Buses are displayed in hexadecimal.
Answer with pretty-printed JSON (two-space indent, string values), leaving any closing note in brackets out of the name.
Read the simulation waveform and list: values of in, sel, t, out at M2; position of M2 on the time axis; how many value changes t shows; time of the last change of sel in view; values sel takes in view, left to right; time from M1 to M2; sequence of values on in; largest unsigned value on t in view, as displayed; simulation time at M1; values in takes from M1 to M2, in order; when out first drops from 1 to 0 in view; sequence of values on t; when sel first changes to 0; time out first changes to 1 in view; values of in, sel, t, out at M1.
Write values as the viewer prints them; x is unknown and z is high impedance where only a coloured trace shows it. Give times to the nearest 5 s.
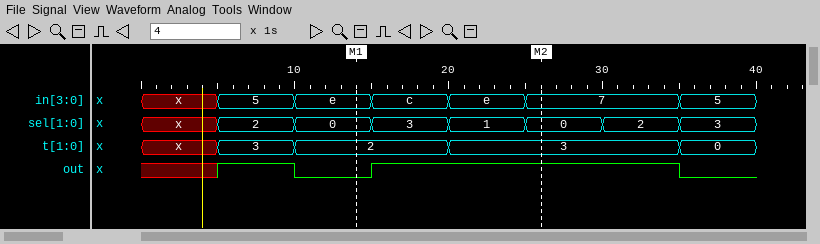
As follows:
{
  "values of in, sel, t, out at M2": "in=7, sel=0, t=3, out=1",
  "position of M2 on the time axis": "25 s",
  "how many value changes t shows": "4",
  "time of the last change of sel in view": "35 s",
  "values sel takes in view, left to right": "x, 2, 0, 3, 1, 0, 2, 3",
  "time from M1 to M2": "10 s",
  "sequence of values on in": "x, 5, e, c, e, 7, 5",
  "largest unsigned value on t in view, as displayed": "3",
  "simulation time at M1": "15 s",
  "values in takes from M1 to M2, in order": "e, c, e, 7",
  "when out first drops from 1 to 0 in view": "10 s",
  "sequence of values on t": "x, 3, 2, 3, 0",
  "when sel first changes to 0": "10 s",
  "time out first changes to 1 in view": "5 s",
  "values of in, sel, t, out at M1": "in=e, sel=0, t=2, out=0"
}
